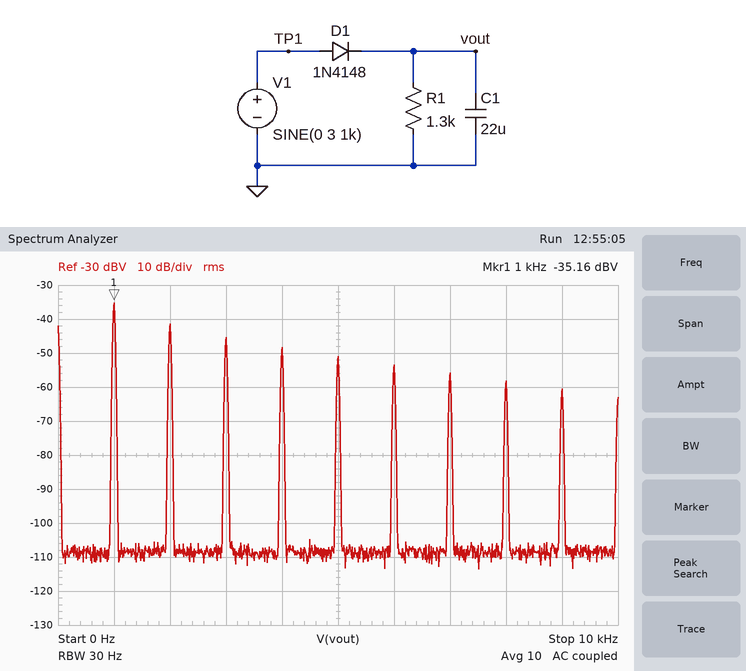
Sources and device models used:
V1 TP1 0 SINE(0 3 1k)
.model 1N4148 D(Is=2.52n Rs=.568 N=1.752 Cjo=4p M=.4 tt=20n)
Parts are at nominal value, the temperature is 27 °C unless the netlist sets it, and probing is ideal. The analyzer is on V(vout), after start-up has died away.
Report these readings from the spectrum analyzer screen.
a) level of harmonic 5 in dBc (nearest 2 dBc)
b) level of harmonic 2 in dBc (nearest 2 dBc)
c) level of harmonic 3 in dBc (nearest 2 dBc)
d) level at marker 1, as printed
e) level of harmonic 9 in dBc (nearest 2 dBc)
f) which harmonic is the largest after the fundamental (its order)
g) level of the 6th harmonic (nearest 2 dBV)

-16 dBc
-6 dBc
-10 dBc
-35.16 dBV
-26 dBc
2
-54 dBV
